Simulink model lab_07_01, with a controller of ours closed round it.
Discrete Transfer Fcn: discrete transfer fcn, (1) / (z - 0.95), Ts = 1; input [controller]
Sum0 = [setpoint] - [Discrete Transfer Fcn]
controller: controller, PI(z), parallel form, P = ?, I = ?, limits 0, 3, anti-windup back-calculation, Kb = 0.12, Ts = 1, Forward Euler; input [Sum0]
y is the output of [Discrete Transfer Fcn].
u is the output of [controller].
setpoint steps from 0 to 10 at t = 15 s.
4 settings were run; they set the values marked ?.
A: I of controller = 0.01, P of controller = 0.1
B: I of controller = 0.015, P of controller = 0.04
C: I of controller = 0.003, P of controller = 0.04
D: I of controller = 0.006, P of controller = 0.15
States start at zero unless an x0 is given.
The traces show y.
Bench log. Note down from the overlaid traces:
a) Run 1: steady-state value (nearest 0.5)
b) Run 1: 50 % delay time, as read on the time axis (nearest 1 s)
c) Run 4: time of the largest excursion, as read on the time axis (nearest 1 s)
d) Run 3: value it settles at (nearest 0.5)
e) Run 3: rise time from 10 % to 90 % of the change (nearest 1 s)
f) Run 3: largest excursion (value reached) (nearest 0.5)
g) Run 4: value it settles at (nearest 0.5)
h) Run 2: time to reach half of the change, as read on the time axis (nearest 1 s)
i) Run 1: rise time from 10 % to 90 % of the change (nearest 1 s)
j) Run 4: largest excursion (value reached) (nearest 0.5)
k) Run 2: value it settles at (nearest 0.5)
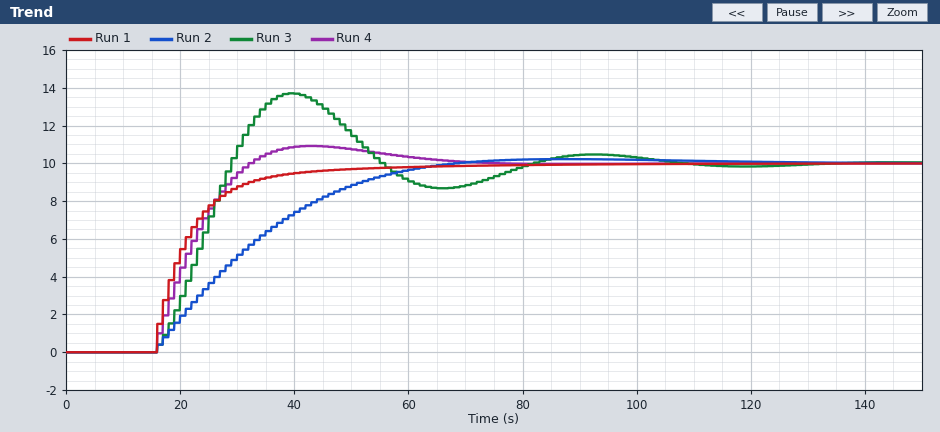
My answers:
10.0
20 s
43 s
10.0
10 s
13.5
10.0
30 s
16 s
11.0
10.0
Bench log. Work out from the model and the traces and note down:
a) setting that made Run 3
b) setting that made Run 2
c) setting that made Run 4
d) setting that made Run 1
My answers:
B
C
A
D
